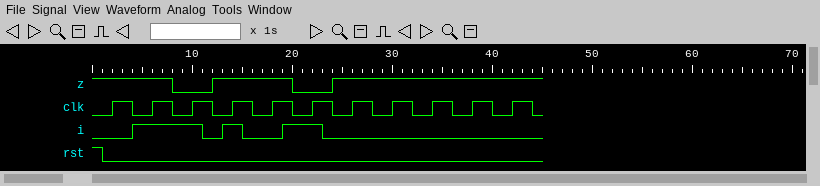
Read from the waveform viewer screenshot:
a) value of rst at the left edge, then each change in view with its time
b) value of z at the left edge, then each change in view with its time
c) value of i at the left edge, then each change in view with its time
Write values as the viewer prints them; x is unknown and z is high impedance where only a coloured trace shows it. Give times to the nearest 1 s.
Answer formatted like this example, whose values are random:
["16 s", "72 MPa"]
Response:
["1, 0 at 1 s", "1, 0 at 8 s, 1 at 12 s, 0 at 20 s, 1 at 24 s", "0, 1 at 4 s, 0 at 11 s, 1 at 13 s, 0 at 15 s, 1 at 19 s, 0 at 23 s"]
